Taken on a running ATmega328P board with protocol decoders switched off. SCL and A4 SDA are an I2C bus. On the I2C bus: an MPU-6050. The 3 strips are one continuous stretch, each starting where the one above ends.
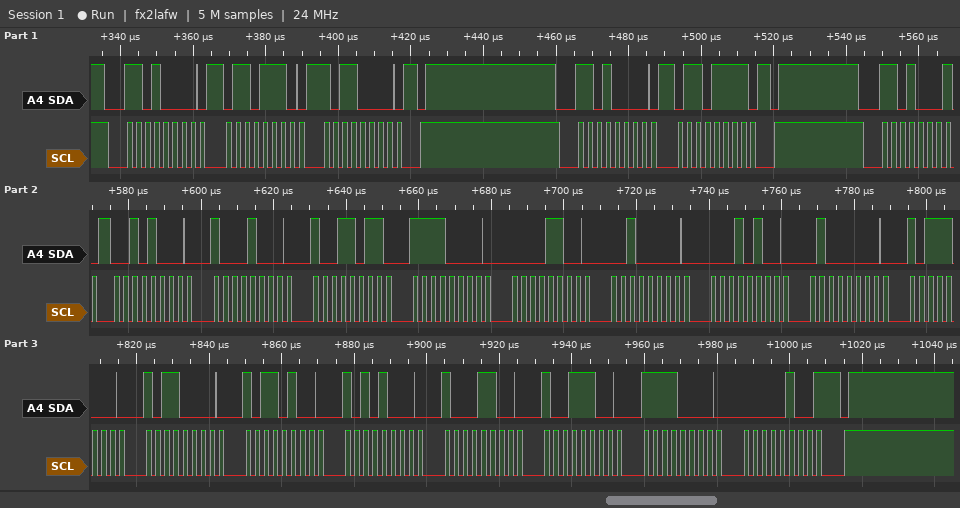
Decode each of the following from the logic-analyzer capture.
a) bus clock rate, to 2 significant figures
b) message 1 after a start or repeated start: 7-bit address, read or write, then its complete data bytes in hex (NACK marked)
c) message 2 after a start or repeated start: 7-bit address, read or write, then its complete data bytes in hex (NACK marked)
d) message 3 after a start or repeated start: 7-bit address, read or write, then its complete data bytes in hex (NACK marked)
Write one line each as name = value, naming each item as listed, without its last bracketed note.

bus clock rate, to 2 significant figures = 400 kHz
message 1 after a start or repeated start: 7-bit address, read or write, then its complete data bytes in hex = 0x68 write: 6E B0
message 2 after a start or repeated start: 7-bit address, read or write, then its complete data bytes in hex = 0x68 write: 6F
message 3 after a start or repeated start: 7-bit address, read or write, then its complete data bytes in hex = 0x68 read: 28 88 9B F0 0C 20 14 40 B8 B0 B4 A8 8C 9C F0 04 NACK
